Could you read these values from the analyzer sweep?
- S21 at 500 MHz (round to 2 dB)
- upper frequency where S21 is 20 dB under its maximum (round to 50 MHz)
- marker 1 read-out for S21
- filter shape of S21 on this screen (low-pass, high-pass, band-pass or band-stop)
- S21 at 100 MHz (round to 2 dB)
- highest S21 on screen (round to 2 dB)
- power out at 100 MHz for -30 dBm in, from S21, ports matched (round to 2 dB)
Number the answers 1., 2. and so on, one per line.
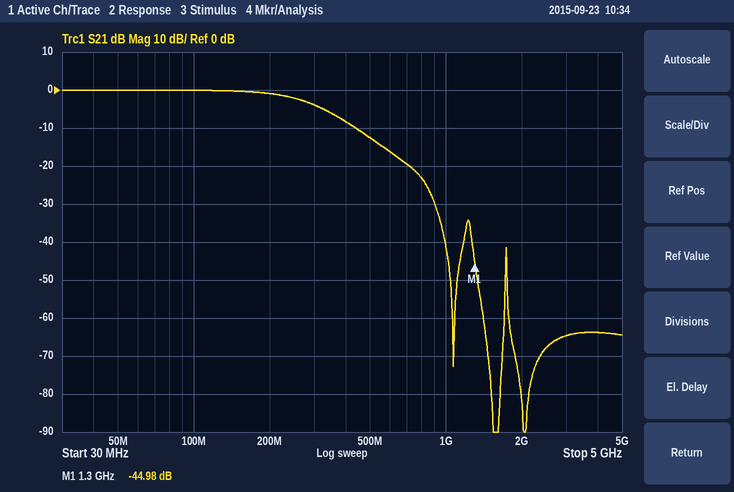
1. -12 dB
2. 700 MHz
3. -44.98 dB
4. low-pass
5. 0 dB
6. 0 dB
7. -30 dBm
